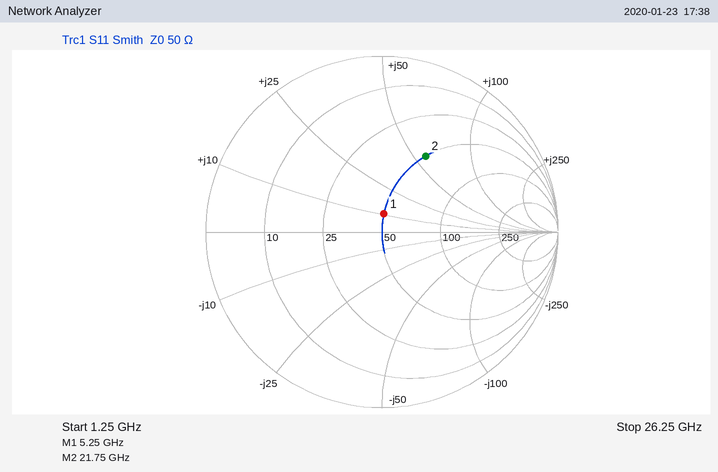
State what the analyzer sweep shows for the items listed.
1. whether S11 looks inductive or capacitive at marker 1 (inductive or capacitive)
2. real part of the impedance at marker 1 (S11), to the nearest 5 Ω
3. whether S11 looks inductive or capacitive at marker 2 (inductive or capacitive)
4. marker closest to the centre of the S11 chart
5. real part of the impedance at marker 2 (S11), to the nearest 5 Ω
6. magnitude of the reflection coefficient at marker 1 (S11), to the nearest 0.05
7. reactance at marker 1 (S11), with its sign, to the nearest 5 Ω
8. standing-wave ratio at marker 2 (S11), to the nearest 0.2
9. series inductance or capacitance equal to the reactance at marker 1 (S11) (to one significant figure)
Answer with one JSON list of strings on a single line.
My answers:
["inductive", "50 Ω", "inductive", "marker 1", "50 Ω", "0.10", "+10 Ω", "3.0", "300 pH"]
